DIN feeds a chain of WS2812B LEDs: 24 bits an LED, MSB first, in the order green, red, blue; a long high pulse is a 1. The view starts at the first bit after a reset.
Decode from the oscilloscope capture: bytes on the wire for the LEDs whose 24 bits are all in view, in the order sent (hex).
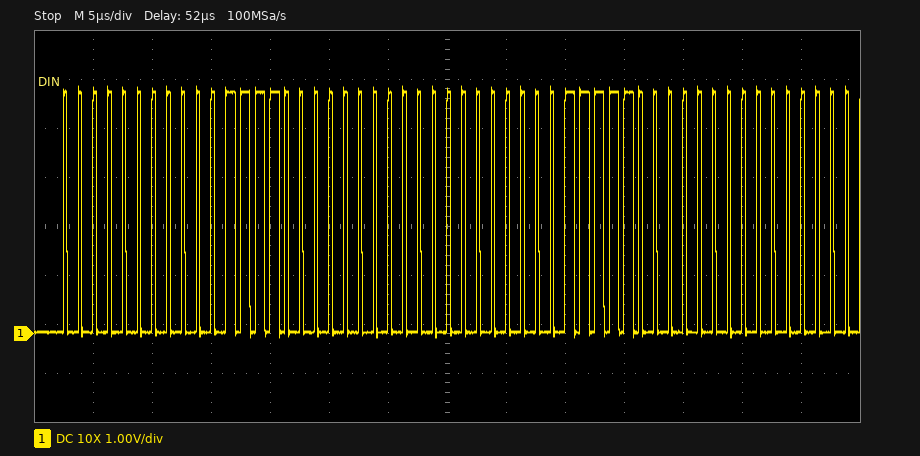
00 1E 00 00 3E 00
